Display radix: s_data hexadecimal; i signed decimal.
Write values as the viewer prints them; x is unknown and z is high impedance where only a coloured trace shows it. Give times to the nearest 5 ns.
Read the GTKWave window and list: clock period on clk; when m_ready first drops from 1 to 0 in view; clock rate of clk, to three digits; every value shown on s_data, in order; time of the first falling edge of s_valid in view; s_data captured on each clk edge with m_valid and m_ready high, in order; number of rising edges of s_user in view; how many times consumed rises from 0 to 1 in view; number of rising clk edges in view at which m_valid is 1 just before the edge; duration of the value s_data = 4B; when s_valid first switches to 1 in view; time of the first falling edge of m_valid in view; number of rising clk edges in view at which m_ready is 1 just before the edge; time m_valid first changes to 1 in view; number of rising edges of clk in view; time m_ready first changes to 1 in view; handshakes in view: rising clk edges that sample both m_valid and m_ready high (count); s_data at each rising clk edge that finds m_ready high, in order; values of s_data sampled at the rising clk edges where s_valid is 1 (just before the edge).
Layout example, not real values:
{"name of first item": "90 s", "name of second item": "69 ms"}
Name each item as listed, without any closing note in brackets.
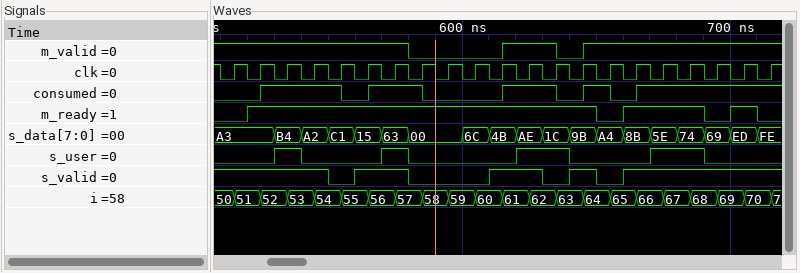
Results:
{"clock period on clk": "10 ns", "when m_ready first drops from 1 to 0 in view": "650 ns", "clock rate of clk, to three digits": "100 MHz", "every value shown on s_data, in order": "A3, B4, A2, C1, 15, 63, 00, 6C, 4B, AE, 1C, 9B, A4, 8B, 5E, 74, 69, ED, FE", "time of the first falling edge of s_valid in view": "550 ns", "s_data captured on each clk edge with m_valid and m_ready high, in order": "A3, B4, A2, C1, 15, 63, AE, 1C, 8B, 5E, 74, ED", "number of rising edges of s_user in view": "4", "how many times consumed rises from 0 to 1 in view": "5", "number of rising clk edges in view at which m_valid is 1 just before the edge": "16", "duration of the value s_data = 4B": "10 ns", "when s_valid first switches to 1 in view": "560 ns", "time of the first falling edge of m_valid in view": "580 ns", "number of rising clk edges in view at which m_ready is 1 just before the edge": "17", "time m_valid first changes to 1 in view": "615 ns", "number of rising edges of clk in view": "21", "time m_ready first changes to 1 in view": "520 ns", "handshakes in view: rising clk edges that sample both m_valid and m_ready high": "12", "s_data at each rising clk edge that finds m_ready high, in order": "A3, B4, A2, C1, 15, 63, 00, 00, 6C, 4B, AE, 1C, 9B, 8B, 5E, 74, ED", "values of s_data sampled at the rising clk edges where s_valid is 1": "A3, A3, B4, A2, 15, 63, 4B, AE, 9B, 8B, 5E, 74, 69, ED, FE"}
